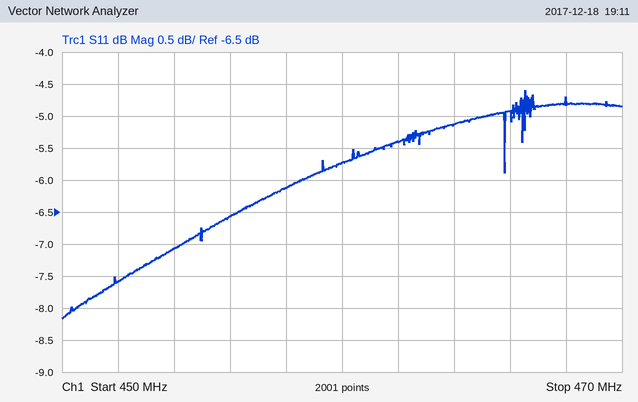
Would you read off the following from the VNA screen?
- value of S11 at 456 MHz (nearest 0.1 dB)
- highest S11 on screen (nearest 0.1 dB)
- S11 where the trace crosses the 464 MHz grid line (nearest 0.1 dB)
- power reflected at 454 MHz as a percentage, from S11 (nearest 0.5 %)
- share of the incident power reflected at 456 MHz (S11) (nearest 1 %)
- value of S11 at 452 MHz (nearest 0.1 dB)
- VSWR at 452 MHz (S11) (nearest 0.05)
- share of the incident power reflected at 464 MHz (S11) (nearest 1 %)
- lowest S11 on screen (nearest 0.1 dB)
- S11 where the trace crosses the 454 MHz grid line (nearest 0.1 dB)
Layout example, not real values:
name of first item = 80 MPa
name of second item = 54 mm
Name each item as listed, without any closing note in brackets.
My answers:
value of S11 at 456 MHz = -6.6 dB
highest S11 on screen = -4.6 dB
S11 where the trace crosses the 464 MHz grid line = -5.1 dB
power reflected at 454 MHz as a percentage, from S11 = 19.5 %
share of the incident power reflected at 456 MHz (S11) = 22 %
value of S11 at 452 MHz = -7.6 dB
VSWR at 452 MHz (S11) = 2.45
share of the incident power reflected at 464 MHz (S11) = 31 %
lowest S11 on screen = -8.2 dB
S11 where the trace crosses the 454 MHz grid line = -7.1 dB
